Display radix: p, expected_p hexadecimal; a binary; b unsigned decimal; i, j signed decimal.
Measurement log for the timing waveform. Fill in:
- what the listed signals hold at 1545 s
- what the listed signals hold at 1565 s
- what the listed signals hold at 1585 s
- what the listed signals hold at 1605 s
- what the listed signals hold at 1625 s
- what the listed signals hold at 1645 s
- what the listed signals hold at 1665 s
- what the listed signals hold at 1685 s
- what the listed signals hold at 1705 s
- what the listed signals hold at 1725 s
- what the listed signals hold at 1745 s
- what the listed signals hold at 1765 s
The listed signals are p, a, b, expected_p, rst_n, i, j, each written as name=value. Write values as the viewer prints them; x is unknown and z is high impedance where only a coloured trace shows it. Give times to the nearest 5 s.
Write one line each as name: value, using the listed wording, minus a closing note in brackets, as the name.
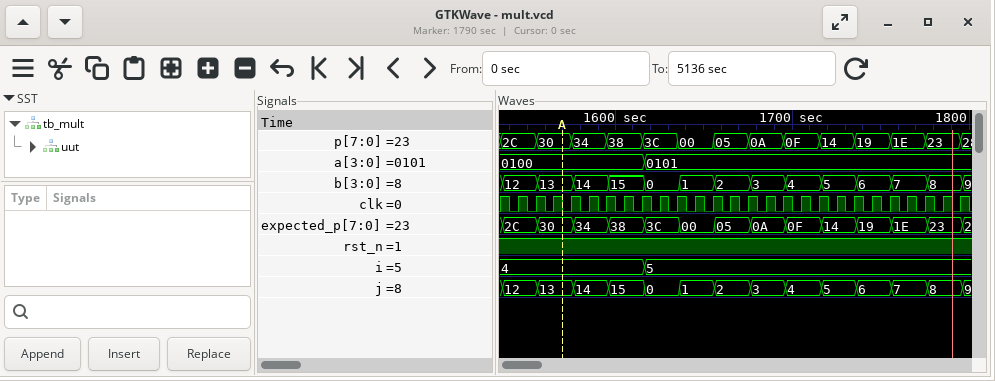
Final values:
what the listed signals hold at 1545 s: p=2C, a=0100, b=12, expected_p=2C, rst_n=1, i=4, j=12
what the listed signals hold at 1565 s: p=30, a=0100, b=13, expected_p=30, rst_n=1, i=4, j=13
what the listed signals hold at 1585 s: p=34, a=0100, b=14, expected_p=34, rst_n=1, i=4, j=14
what the listed signals hold at 1605 s: p=38, a=0100, b=15, expected_p=38, rst_n=1, i=4, j=15
what the listed signals hold at 1625 s: p=3C, a=0101, b=0, expected_p=3C, rst_n=1, i=5, j=0
what the listed signals hold at 1645 s: p=00, a=0101, b=1, expected_p=00, rst_n=1, i=5, j=1
what the listed signals hold at 1665 s: p=05, a=0101, b=2, expected_p=05, rst_n=1, i=5, j=2
what the listed signals hold at 1685 s: p=0A, a=0101, b=3, expected_p=0A, rst_n=1, i=5, j=3
what the listed signals hold at 1705 s: p=0F, a=0101, b=4, expected_p=0F, rst_n=1, i=5, j=4
what the listed signals hold at 1725 s: p=14, a=0101, b=5, expected_p=14, rst_n=1, i=5, j=5
what the listed signals hold at 1745 s: p=19, a=0101, b=6, expected_p=19, rst_n=1, i=5, j=6
what the listed signals hold at 1765 s: p=1E, a=0101, b=7, expected_p=1E, rst_n=1, i=5, j=7
